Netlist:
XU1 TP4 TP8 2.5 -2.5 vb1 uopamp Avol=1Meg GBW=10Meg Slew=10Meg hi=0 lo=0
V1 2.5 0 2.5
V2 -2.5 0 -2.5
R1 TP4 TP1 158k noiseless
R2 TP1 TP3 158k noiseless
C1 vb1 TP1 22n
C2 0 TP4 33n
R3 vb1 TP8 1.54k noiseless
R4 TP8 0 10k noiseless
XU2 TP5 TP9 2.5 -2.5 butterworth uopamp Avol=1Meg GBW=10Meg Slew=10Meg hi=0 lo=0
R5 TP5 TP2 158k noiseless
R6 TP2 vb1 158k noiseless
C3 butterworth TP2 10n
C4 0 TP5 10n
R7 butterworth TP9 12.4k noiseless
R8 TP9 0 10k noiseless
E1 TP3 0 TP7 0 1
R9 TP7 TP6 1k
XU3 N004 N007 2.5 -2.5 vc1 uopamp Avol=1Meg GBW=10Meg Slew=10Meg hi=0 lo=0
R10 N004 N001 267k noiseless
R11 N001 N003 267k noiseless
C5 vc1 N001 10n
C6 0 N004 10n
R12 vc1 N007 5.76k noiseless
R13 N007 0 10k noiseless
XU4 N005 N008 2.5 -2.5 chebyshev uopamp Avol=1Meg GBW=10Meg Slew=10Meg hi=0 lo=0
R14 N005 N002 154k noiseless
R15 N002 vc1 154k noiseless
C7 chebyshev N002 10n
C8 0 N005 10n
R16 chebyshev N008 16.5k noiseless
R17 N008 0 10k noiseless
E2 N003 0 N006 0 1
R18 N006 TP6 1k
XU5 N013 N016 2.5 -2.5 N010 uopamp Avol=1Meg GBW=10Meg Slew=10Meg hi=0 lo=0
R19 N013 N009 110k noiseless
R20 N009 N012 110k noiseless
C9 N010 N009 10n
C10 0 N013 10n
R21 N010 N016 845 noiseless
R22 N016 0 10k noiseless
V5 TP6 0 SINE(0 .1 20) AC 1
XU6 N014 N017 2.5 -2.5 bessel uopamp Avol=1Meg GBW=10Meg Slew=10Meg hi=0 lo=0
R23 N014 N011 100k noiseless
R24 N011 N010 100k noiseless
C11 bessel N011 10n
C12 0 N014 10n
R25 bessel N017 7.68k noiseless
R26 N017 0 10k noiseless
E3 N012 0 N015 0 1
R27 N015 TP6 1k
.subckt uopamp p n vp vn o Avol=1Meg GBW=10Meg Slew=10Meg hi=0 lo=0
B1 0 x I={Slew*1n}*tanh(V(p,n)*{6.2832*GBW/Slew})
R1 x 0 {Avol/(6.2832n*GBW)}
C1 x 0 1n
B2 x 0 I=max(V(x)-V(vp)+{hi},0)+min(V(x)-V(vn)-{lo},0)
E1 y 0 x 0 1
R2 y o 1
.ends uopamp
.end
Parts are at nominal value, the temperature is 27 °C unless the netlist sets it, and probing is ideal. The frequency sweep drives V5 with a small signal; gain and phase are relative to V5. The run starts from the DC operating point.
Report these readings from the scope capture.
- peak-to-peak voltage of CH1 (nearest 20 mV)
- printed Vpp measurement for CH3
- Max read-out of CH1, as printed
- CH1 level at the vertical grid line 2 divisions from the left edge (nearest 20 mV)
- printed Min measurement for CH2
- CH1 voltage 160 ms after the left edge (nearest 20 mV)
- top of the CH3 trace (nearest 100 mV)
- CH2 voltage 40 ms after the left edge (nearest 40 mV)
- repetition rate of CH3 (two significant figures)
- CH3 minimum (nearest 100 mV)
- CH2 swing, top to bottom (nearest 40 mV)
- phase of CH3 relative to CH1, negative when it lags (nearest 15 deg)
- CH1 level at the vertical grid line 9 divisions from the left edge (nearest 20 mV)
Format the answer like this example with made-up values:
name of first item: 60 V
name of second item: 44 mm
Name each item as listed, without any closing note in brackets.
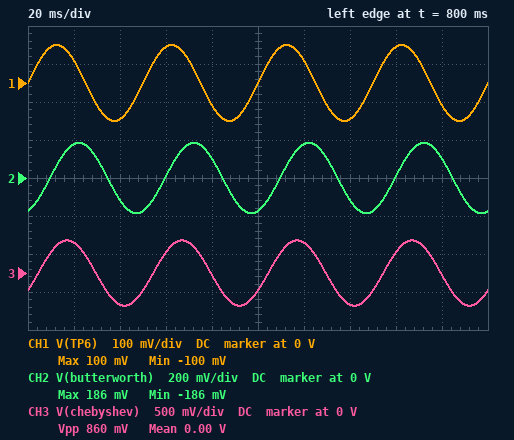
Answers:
peak-to-peak voltage of CH1: 200 mV
printed Vpp measurement for CH3: 860 mV
Max read-out of CH1, as printed: 100 mV
CH1 level at the vertical grid line 2 divisions from the left edge: -100 mV
printed Min measurement for CH2: -186 mV
CH1 voltage 160 ms after the left edge: 100 mV
top of the CH3 trace: 400 mV
CH2 voltage 40 ms after the left edge: -120 mV
repetition rate of CH3: 20 Hz
CH3 minimum: -400 mV
CH2 swing, top to bottom: 360 mV
phase of CH3 relative to CH1, negative when it lags: -30 deg
CH1 level at the vertical grid line 9 divisions from the left edge: -60 mV
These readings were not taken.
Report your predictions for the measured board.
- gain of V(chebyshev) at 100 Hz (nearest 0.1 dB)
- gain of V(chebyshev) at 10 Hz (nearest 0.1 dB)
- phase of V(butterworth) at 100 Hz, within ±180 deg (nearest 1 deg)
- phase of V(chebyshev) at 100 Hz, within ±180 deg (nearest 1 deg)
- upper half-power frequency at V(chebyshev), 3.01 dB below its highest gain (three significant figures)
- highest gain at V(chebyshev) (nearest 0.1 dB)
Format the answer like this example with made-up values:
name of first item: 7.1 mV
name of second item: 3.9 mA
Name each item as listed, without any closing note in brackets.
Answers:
gain of V(chebyshev) at 100 Hz: 12.1 dB
gain of V(chebyshev) at 10 Hz: 12.5 dB
phase of V(butterworth) at 100 Hz, within ±180 deg: 136 deg
phase of V(chebyshev) at 100 Hz, within ±180 deg: 153 deg
upper half-power frequency at V(chebyshev), 3.01 dB below its highest gain: 109 Hz
highest gain at V(chebyshev): 12.9 dB
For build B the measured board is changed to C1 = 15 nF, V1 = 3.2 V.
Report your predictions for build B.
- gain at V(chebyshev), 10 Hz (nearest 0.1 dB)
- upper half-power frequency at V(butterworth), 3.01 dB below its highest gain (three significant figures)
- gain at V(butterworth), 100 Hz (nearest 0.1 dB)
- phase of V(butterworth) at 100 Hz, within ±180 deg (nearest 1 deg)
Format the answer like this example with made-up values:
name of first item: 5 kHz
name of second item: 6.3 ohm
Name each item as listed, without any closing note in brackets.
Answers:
gain at V(chebyshev), 10 Hz: 12.5 dB
upper half-power frequency at V(butterworth), 3.01 dB below its highest gain: 18.8 Hz
gain at V(butterworth), 100 Hz: -6.7 dB
phase of V(butterworth) at 100 Hz, within ±180 deg: 150 deg
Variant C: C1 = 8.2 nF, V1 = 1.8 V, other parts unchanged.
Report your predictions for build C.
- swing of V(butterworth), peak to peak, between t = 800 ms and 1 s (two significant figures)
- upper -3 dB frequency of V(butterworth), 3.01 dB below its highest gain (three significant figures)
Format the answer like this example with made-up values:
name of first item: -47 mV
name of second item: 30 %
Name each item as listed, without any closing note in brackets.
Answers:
swing of V(butterworth), peak to peak, between t = 800 ms and 1 s: 340 mV
upper -3 dB frequency of V(butterworth), 3.01 dB below its highest gain: 17.3 Hz
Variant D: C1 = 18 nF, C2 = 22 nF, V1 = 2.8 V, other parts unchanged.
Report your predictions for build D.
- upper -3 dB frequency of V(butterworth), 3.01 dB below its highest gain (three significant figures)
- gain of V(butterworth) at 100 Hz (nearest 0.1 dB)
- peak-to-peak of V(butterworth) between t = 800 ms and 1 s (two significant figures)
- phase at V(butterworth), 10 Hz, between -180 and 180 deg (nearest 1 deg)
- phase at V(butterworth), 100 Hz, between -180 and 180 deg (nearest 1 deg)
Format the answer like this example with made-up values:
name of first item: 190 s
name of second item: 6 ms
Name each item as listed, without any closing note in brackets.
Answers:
upper -3 dB frequency of V(butterworth), 3.01 dB below its highest gain: 35.7 Hz
gain of V(butterworth) at 100 Hz: -3.3 dB
peak-to-peak of V(butterworth) between t = 800 ms and 1 s: 450 mV
phase at V(butterworth), 10 Hz, between -180 and 180 deg: -27 deg
phase at V(butterworth), 100 Hz, between -180 and 180 deg: 146 deg
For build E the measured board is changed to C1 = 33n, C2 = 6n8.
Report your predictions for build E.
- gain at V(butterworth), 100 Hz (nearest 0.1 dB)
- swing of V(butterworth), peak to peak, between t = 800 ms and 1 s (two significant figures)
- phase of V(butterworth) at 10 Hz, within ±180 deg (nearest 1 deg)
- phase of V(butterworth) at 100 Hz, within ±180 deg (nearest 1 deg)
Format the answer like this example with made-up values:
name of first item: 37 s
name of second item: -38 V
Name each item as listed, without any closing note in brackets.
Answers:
gain at V(butterworth), 100 Hz: 7.3 dB
swing of V(butterworth), peak to peak, between t = 800 ms and 1 s: 570 mV
phase of V(butterworth) at 10 Hz, within ±180 deg: -9 deg
phase of V(butterworth) at 100 Hz, within ±180 deg: 126 deg
